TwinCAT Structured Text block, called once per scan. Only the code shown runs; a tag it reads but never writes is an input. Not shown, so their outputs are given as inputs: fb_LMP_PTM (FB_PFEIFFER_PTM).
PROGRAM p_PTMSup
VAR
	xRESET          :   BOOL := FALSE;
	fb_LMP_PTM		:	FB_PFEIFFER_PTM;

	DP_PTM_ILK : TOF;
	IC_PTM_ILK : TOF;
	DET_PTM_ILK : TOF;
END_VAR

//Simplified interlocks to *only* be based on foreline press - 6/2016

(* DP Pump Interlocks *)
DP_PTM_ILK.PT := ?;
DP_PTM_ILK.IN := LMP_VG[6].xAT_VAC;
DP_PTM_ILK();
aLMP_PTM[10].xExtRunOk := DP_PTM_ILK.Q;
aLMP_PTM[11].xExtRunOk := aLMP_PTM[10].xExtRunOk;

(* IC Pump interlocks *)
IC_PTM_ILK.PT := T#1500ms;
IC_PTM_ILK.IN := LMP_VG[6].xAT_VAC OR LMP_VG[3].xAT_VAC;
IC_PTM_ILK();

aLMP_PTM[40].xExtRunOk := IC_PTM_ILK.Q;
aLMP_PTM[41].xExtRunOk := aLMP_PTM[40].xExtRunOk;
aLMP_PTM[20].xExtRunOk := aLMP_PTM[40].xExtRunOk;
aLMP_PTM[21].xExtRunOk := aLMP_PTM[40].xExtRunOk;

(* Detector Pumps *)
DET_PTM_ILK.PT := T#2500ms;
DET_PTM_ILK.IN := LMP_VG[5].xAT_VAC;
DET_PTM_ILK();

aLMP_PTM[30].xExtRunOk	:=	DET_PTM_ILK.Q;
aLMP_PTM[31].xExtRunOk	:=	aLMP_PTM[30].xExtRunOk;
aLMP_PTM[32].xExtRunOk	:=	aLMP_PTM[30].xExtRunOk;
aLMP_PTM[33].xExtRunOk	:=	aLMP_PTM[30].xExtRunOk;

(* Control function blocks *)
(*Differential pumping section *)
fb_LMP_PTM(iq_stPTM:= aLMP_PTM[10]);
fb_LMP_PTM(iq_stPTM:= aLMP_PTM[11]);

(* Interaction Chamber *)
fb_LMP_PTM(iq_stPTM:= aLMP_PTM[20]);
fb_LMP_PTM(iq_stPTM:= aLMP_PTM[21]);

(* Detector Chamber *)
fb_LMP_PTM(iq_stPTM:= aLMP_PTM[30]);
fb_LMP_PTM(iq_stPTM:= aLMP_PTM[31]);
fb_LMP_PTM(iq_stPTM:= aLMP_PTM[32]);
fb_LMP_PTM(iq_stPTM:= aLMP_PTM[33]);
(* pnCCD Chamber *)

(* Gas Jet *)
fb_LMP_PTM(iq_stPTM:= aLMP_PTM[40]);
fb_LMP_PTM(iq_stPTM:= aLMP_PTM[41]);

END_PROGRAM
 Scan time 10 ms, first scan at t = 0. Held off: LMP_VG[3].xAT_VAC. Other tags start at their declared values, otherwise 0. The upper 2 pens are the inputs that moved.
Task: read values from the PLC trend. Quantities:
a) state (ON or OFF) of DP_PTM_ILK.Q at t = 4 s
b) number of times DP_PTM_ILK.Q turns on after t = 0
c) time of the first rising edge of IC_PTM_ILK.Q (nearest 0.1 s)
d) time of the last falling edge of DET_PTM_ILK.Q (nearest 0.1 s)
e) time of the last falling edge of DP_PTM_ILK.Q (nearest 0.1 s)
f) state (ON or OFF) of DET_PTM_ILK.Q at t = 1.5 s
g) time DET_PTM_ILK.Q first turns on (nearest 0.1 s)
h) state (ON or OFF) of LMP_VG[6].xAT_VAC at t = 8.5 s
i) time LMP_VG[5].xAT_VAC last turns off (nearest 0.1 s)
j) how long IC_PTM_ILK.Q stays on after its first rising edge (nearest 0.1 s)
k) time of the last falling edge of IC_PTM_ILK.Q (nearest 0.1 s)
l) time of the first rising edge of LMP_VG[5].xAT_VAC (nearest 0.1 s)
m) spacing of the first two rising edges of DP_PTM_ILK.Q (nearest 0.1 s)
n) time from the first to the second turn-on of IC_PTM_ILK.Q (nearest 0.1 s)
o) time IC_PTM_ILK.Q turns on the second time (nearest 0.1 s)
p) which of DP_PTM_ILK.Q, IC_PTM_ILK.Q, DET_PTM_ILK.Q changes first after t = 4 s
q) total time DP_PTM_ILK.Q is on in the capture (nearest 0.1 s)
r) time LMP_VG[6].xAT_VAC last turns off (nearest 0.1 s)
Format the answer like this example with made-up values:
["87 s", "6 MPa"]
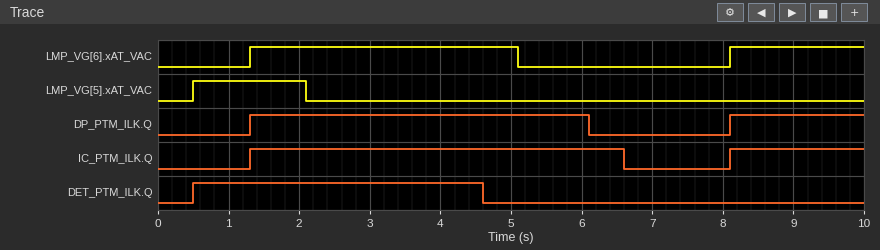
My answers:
["ON", "2", "1.3 s", "4.6 s", "6.1 s", "ON", "0.5 s", "ON", "2.1 s", "5.3 s", "6.6 s", "0.5 s", "6.8 s", "6.8 s", "8.1 s", "DET_PTM_ILK.Q", "6.7 s", "5.1 s"]
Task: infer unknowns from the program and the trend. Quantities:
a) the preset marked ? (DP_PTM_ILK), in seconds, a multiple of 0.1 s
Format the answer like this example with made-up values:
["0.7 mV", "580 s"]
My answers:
["1.0 s"]
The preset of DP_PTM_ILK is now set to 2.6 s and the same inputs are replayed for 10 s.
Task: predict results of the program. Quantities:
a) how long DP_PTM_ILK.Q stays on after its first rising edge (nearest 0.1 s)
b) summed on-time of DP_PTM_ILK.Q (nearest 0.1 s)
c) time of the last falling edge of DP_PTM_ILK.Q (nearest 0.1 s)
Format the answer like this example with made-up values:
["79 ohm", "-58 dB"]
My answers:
["6.4 s", "8.3 s", "7.7 s"]
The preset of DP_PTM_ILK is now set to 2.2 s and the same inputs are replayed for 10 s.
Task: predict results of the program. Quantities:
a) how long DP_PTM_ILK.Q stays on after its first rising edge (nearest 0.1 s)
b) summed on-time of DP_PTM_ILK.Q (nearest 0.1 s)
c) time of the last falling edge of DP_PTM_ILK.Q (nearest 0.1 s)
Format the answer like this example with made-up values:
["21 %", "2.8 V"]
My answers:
["6.0 s", "7.9 s", "7.3 s"]
